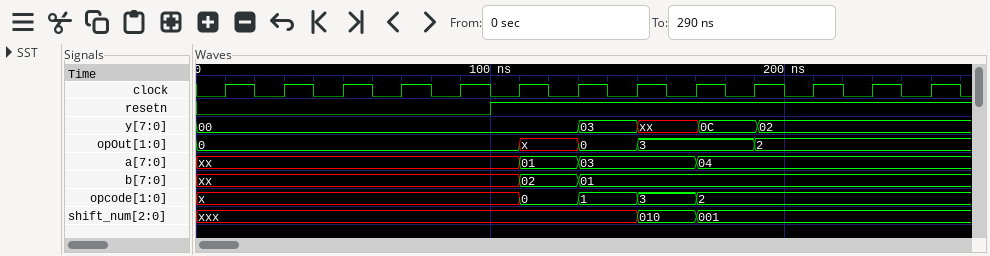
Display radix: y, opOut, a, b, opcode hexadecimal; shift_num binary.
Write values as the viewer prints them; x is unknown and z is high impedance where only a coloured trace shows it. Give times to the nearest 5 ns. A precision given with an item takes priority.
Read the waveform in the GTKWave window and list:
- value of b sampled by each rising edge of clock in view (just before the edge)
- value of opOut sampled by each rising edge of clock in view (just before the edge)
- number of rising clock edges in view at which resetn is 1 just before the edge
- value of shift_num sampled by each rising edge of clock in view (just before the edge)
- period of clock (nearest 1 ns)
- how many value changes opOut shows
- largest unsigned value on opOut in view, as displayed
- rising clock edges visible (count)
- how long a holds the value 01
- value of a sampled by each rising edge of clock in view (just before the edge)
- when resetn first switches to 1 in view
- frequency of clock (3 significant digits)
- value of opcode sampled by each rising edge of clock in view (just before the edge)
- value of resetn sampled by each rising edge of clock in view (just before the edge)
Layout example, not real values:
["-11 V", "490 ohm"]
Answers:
["xx, xx, xx, xx, xx, xx, 02, 01, 01, 01, 01, 01, 01", "0, 0, 0, 0, 0, 0, x, 0, 3, 3, 2, 2, 2", "8", "xxx, xxx, xxx, xxx, xxx, xxx, xxx, xxx, 010, 001, 001, 001, 001", "20 ns", "4", "3", "13", "20 ns", "xx, xx, xx, xx, xx, xx, 01, 03, 03, 04, 04, 04, 04", "100 ns", "50.0 MHz", "x, x, x, x, x, x, 0, 1, 3, 2, 2, 2, 2", "0 0 0 0 0 1 1 1 1 1 1 1 1"]
